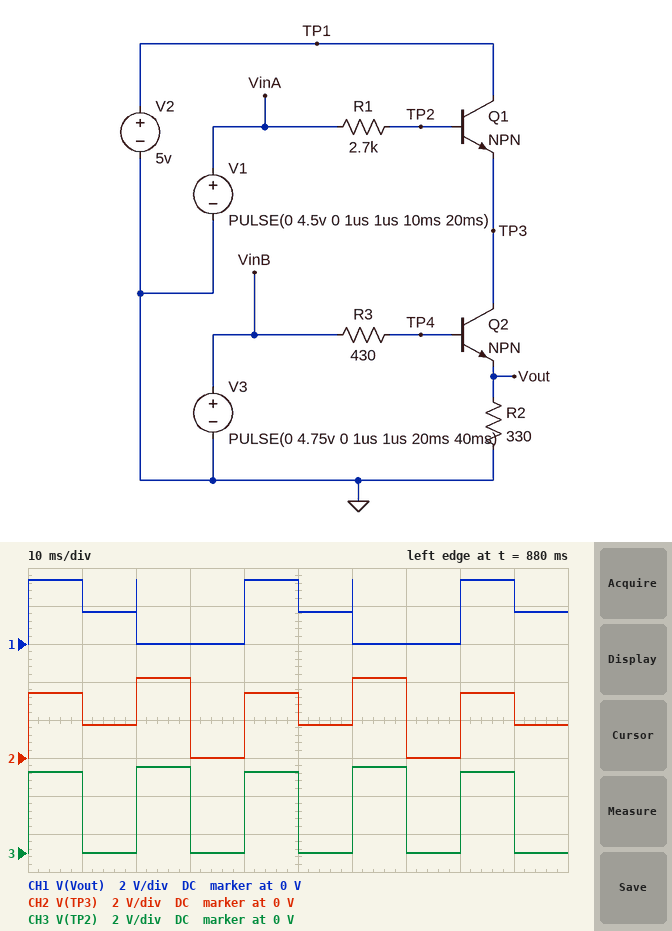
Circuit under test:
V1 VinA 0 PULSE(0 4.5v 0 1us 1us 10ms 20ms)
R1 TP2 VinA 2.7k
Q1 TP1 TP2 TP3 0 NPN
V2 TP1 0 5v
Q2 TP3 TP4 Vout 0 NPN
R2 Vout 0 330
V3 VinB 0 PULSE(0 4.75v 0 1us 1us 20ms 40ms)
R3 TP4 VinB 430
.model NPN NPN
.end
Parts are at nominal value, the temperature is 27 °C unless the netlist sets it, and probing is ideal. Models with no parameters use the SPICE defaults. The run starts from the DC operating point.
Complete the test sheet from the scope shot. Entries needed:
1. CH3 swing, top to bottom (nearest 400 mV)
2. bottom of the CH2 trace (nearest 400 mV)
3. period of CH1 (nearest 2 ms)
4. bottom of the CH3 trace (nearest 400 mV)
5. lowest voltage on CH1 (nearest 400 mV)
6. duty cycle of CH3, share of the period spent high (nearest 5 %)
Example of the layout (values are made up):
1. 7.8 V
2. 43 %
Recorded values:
1. 4.4 V
2. 0 V
3. 40 ms
4. 0 V
5. 0 V
6. 50 %
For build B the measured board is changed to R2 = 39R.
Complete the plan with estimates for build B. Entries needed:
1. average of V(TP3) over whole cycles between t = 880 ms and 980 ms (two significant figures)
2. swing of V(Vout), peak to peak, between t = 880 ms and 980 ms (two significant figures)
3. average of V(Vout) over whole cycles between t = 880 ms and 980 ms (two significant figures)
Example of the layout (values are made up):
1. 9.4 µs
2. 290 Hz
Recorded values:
1. 1.6 V
2. 2.2 V
3. 620 mV
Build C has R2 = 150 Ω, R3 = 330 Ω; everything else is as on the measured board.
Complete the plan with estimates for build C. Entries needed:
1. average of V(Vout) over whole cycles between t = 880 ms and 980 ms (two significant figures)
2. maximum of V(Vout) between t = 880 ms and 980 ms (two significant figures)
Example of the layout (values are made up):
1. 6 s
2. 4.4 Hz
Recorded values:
1. 1.1 V
2. 3.1 V
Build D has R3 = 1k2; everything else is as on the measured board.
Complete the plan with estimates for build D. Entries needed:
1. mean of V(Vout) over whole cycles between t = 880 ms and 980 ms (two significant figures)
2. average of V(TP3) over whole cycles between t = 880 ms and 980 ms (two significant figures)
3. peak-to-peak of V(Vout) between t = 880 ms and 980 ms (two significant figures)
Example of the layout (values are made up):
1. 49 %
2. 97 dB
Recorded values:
1. 1.0 V
2. 2.1 V
3. 3.3 V
